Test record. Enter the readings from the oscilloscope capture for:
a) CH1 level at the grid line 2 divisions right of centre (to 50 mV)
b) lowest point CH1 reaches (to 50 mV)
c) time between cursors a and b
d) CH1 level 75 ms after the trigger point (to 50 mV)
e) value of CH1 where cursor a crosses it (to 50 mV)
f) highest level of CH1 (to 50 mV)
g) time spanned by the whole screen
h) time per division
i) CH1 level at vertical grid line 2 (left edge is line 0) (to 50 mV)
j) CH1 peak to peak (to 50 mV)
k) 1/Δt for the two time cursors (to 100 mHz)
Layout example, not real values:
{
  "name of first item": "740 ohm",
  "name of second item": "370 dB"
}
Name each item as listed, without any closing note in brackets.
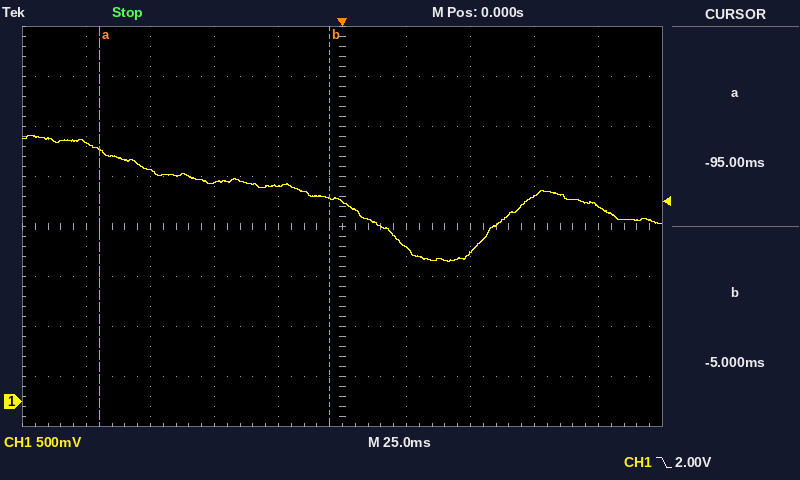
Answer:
{
  "CH1 level at the grid line 2 divisions right of centre": "1.50 V",
  "lowest point CH1 reaches": "1.40 V",
  "time between cursors a and b": "90.0 ms",
  "CH1 level 75 ms after the trigger point": "2.05 V",
  "value of CH1 where cursor a crosses it": "2.50 V",
  "highest level of CH1": "2.65 V",
  "time spanned by the whole screen": "250 ms",
  "time per division": "25 ms",
  "CH1 level at vertical grid line 2 (left edge is line 0)": "2.30 V",
  "CH1 peak to peak": "1.25 V",
  "1/Δt for the two time cursors": "11.1 Hz"
}
